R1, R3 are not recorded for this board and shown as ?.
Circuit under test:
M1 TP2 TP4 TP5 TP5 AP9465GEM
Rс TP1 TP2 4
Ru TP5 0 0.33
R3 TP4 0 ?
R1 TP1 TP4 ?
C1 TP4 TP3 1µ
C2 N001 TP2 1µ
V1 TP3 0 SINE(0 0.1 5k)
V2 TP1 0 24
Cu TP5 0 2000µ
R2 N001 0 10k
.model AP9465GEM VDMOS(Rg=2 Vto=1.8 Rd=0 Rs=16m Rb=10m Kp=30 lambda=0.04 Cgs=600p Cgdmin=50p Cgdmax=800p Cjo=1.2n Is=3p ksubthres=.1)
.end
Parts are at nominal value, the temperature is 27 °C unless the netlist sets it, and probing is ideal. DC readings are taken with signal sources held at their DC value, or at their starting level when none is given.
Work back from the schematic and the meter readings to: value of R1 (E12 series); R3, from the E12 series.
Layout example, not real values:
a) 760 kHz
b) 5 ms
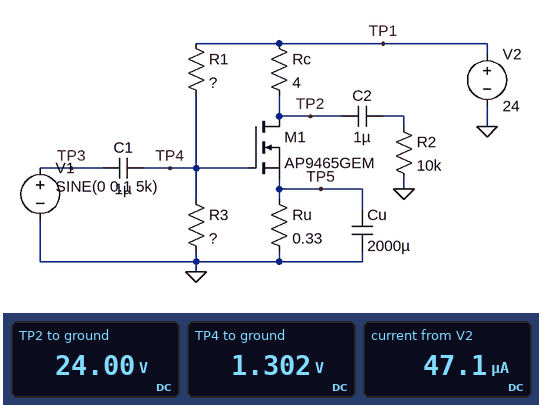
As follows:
a) 680 kΩ
b) 39 kΩ
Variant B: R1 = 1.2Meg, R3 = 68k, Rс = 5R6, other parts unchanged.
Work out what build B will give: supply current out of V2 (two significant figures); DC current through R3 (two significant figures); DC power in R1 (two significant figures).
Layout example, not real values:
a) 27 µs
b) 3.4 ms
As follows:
a) 29 µA
b) 19 µA
c) 430 µW
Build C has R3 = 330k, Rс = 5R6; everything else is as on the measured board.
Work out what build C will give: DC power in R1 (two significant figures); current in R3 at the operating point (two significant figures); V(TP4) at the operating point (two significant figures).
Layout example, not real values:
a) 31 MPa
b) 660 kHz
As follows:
a) 380 µW
b) 24 µA
c) 7.8 V
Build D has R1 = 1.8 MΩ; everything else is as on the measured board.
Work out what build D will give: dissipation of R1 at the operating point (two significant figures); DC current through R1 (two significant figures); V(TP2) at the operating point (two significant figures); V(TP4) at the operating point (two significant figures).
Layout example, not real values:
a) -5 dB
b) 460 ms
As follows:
a) 310 µW
b) 13 µA
c) 24 V
d) 510 mV
